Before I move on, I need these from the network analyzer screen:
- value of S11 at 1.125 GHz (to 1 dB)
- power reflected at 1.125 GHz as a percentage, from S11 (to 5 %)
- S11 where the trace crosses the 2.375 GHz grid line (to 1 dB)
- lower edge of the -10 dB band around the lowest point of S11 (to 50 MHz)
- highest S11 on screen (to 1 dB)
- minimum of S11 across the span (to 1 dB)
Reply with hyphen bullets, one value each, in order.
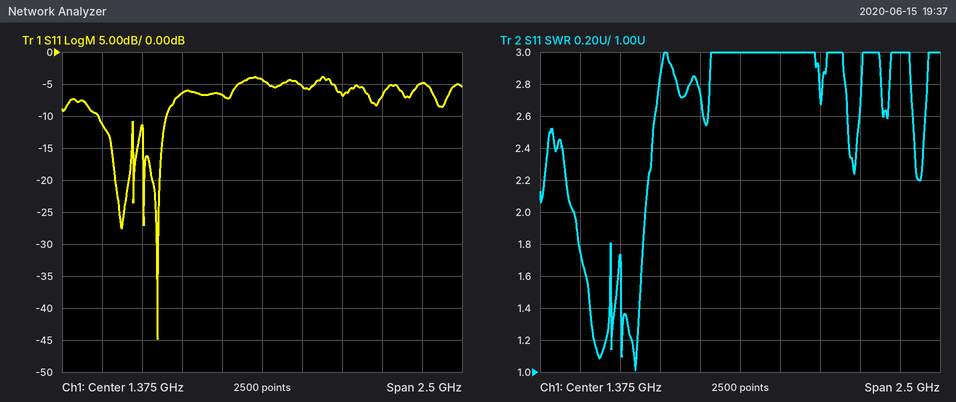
- -7 dB
- 20 %
- -5 dB
- 350 MHz
- -4 dB
- -45 dB
